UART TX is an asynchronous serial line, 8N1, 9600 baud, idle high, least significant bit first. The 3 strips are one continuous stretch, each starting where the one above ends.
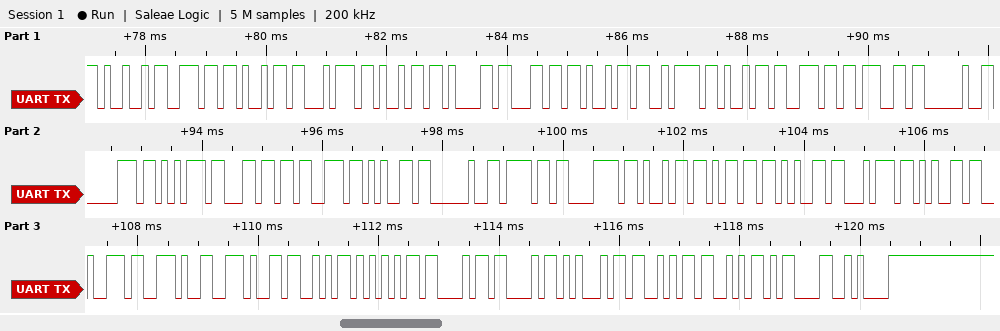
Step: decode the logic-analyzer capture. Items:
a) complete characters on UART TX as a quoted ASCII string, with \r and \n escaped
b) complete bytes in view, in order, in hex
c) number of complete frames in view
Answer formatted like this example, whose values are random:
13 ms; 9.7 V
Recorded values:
"Initializing pulse oximeter..SUCCESS\r\n"; 0x49 0x6E 0x69 0x74 0x69 0x61 0x6C 0x69 0x7A 0x69 0x6E 0x67 0x20 0x70 0x75 0x6C 0x73 0x65 0x20 0x6F 0x78 0x69 0x6D 0x65 0x74 0x65 0x72 0x2E 0x2E 0x53 0x55 0x43 0x43 0x45 0x53 0x53 0x0D 0x0A; 38
